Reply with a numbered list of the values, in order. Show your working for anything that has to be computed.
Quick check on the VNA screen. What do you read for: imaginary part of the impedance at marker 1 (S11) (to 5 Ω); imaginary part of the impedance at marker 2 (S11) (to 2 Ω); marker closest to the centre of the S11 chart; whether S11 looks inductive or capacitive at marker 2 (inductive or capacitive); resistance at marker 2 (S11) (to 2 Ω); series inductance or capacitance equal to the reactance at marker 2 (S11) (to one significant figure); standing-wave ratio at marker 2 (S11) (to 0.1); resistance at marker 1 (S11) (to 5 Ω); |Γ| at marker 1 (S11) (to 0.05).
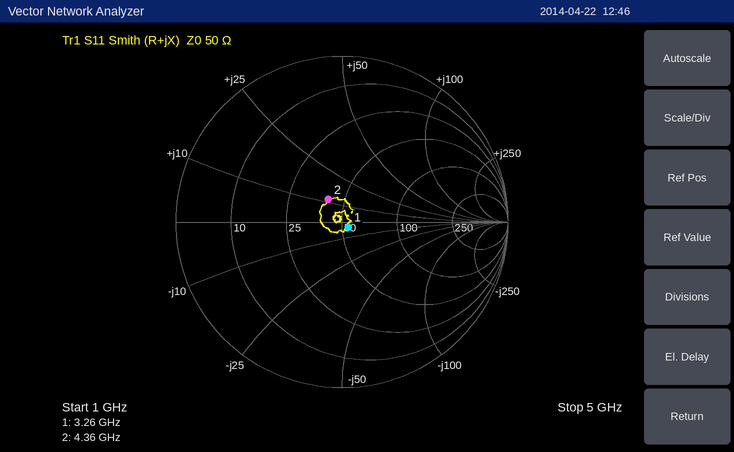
1. -5 Ω
2. +12 Ω
3. marker 1
4. inductive
5. 40 Ω
6. L = 12 Ω/(2π × 4.36 GHz) ≈ 438 pH, so 400 pH to one significant figure
7. 1.4
8. 55 Ω
9. 0.05
